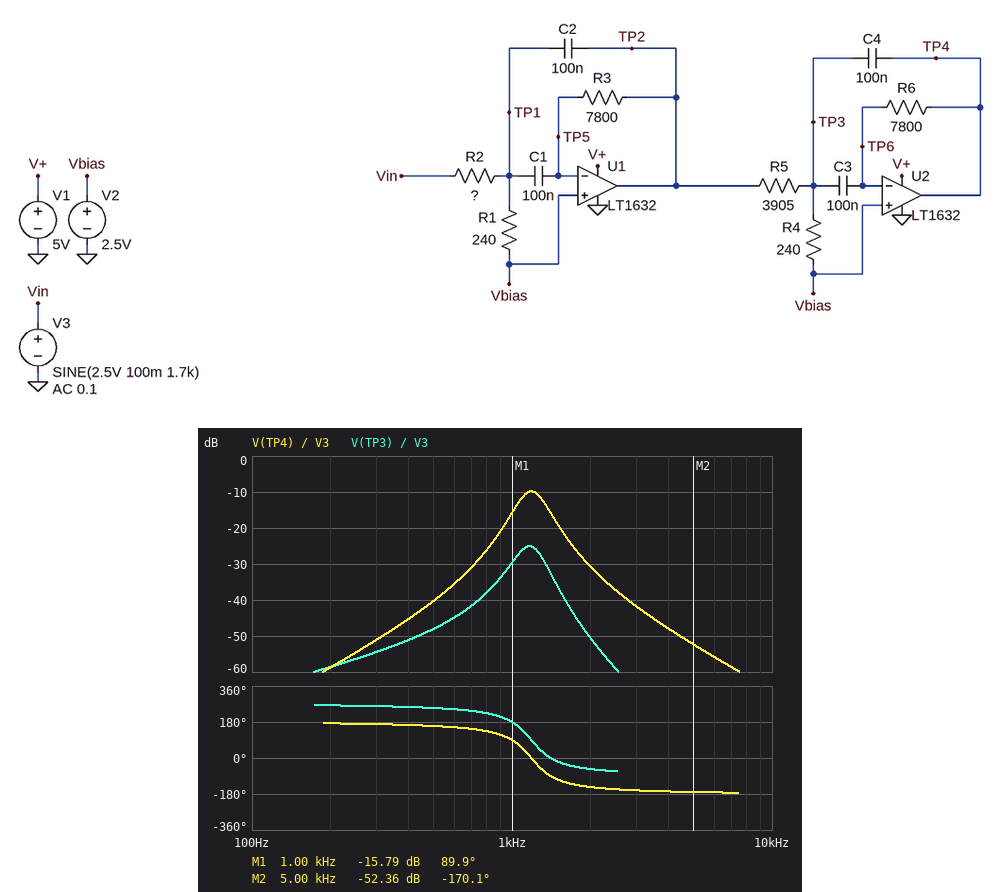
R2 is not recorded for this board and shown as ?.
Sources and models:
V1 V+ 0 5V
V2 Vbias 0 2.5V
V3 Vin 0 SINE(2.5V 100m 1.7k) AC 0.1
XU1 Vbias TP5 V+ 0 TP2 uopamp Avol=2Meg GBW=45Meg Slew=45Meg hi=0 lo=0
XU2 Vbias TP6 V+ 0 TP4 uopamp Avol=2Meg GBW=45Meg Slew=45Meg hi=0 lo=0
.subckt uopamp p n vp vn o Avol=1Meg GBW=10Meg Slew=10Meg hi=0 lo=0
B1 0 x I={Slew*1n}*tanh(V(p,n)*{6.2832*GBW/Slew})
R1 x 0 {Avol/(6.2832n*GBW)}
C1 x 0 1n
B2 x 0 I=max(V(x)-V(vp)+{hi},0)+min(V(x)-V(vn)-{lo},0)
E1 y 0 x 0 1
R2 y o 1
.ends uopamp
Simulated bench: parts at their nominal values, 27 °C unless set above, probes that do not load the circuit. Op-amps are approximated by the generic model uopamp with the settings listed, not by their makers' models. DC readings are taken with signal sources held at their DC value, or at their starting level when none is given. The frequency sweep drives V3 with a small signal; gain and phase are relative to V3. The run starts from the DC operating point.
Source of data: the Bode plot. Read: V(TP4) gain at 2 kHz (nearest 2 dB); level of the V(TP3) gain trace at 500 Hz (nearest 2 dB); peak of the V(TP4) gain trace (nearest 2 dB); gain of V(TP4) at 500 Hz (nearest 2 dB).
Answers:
-30 dB
-48 dB
-10 dB
-40 dB
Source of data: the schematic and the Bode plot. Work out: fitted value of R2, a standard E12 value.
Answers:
12 kΩ
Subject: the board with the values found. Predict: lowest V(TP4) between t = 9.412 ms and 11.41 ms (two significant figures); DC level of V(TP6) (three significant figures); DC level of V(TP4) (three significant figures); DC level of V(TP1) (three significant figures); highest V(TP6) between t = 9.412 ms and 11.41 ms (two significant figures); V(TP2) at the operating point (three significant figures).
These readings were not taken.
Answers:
2.5 V
2.50 V
2.50 V
2.50 V
2.5 V
2.50 V
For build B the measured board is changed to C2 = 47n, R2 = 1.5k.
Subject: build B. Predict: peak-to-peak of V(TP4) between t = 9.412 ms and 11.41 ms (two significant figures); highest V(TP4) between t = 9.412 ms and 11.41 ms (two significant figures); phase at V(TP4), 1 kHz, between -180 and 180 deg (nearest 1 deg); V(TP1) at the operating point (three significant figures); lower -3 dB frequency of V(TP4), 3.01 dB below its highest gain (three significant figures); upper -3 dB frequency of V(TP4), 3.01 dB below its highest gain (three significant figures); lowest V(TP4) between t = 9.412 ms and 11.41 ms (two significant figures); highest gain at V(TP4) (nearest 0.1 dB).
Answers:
280 mV
2.6 V
122 deg
2.50 V
1.11 kHz
1.97 kHz
2.4 V
3.1 dB
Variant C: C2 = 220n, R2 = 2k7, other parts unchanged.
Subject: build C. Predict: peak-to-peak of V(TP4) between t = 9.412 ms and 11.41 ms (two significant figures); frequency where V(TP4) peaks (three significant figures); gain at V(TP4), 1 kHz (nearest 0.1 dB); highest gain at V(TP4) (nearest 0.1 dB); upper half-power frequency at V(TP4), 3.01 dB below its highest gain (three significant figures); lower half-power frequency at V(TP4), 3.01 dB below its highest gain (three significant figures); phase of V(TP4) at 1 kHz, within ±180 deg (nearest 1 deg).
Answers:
17 mV
1.08 kHz
-7.7 dB
-7.6 dB
1.29 kHz
768 Hz
-1 deg
